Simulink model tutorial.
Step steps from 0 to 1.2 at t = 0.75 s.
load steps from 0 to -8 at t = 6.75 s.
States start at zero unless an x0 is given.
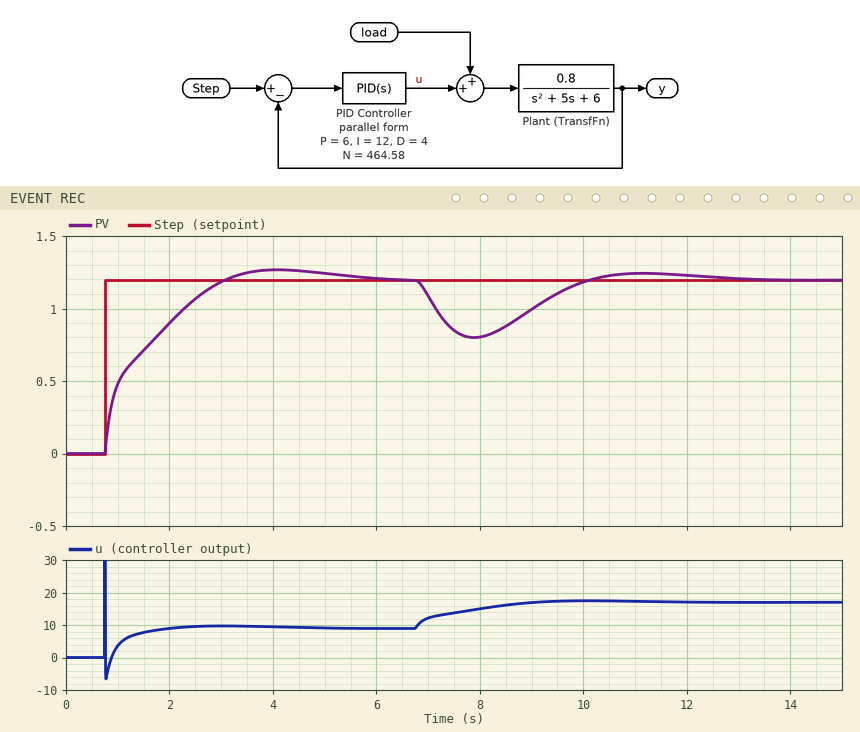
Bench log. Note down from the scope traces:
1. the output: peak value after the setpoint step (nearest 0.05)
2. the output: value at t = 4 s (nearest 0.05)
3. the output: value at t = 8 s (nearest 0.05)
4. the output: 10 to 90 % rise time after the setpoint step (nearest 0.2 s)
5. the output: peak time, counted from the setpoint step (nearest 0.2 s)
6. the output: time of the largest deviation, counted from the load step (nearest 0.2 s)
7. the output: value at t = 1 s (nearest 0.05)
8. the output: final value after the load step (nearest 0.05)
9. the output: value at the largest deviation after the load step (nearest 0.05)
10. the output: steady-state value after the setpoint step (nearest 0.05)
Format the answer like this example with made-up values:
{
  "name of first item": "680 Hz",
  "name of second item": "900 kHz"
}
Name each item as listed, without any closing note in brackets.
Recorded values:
{
  "the output: peak value after the setpoint step": "1.25",
  "the output: value at t = 4 s": "1.25",
  "the output: value at t = 8 s": "0.80",
  "the output: 10 to 90 % rise time after the setpoint step": "1.8 s",
  "the output: peak time, counted from the setpoint step": "3.4 s",
  "the output: time of the largest deviation, counted from the load step": "1.2 s",
  "the output: value at t = 1 s": "0.50",
  "the output: final value after the load step": "1.20",
  "the output: value at the largest deviation after the load step": "0.80",
  "the output: steady-state value after the setpoint step": "1.20"
}
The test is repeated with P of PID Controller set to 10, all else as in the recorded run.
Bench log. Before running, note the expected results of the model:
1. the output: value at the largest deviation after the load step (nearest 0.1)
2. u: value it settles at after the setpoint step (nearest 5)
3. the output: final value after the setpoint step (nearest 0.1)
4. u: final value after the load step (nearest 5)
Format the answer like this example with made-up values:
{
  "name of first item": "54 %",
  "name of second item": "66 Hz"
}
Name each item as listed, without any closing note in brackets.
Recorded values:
{
  "the output: value at the largest deviation after the load step": "0.9",
  "u: value it settles at after the setpoint step": "10",
  "the output: final value after the setpoint step": "1.2",
  "u: final value after the load step": "15"
}
